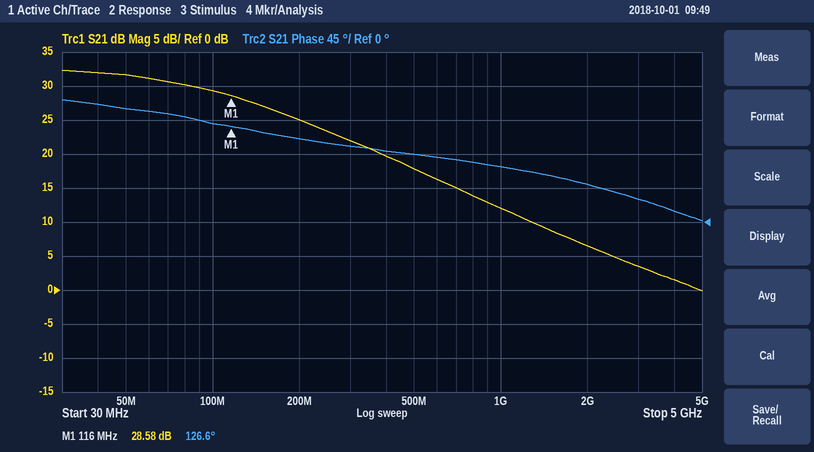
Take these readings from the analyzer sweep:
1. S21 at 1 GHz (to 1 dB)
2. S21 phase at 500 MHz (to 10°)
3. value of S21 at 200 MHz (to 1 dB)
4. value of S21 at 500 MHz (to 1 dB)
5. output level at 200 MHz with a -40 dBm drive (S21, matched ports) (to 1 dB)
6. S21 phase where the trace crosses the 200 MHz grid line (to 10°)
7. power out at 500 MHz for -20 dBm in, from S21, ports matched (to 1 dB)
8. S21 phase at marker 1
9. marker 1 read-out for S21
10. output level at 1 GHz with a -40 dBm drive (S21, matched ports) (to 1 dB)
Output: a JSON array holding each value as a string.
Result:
["12 dB", "90°", "25 dB", "18 dB", "-15 dBm", "110°", "-2 dBm", "126.6°", "28.58 dB", "-28 dBm"]
